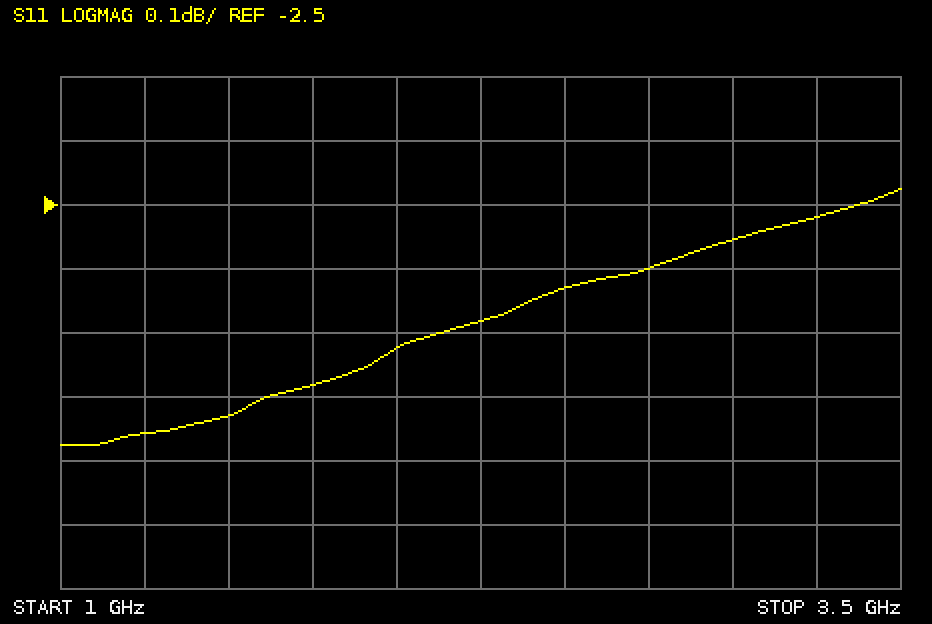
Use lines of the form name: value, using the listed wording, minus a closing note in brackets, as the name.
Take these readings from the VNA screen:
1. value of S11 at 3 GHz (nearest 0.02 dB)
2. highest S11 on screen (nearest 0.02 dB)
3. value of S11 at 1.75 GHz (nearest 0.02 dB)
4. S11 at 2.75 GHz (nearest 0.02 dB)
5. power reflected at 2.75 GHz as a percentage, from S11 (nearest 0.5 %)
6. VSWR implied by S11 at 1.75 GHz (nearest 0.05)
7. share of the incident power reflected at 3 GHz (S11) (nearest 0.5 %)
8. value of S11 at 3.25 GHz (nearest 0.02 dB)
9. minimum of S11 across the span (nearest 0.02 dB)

value of S11 at 3 GHz: -2.56 dB
highest S11 on screen: -2.48 dB
value of S11 at 1.75 GHz: -2.78 dB
S11 at 2.75 GHz: -2.60 dB
power reflected at 2.75 GHz as a percentage, from S11: 55.0 %
VSWR implied by S11 at 1.75 GHz: 6.30
share of the incident power reflected at 3 GHz (S11): 55.5 %
value of S11 at 3.25 GHz: -2.52 dB
minimum of S11 across the span: -2.88 dB
